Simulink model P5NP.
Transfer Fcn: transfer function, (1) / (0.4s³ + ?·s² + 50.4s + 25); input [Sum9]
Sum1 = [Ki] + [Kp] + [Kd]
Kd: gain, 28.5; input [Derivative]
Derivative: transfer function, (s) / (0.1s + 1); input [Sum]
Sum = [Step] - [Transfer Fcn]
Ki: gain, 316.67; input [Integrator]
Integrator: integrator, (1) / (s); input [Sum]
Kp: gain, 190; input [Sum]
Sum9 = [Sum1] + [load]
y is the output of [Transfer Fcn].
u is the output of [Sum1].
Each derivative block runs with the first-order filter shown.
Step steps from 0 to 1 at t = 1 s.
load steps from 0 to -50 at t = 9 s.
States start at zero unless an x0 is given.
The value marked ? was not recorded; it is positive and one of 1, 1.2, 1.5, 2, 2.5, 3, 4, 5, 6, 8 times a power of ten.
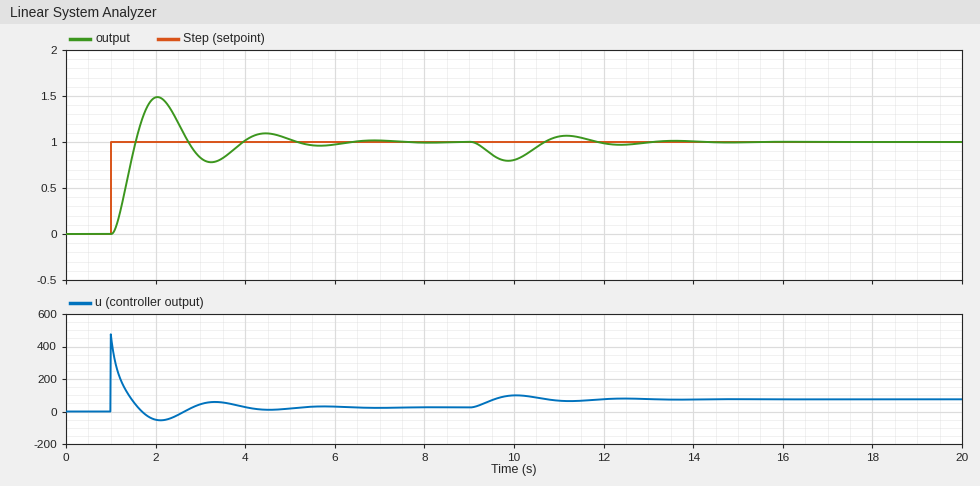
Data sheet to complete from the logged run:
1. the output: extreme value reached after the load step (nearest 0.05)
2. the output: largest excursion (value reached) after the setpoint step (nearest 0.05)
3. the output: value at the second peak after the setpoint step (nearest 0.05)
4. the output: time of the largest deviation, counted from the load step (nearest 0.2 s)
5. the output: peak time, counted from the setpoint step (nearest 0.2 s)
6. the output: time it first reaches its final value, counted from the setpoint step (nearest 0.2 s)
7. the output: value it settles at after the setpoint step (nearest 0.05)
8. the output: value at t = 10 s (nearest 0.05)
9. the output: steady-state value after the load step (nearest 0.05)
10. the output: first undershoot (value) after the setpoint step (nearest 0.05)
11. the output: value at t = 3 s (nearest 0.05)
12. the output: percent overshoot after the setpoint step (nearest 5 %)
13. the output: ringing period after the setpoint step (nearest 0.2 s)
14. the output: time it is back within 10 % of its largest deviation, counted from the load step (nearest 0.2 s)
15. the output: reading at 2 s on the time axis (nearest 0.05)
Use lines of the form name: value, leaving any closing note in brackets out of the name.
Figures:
the output: extreme value reached after the load step: 0.80
the output: largest excursion (value reached) after the setpoint step: 1.50
the output: value at the second peak after the setpoint step: 1.10
the output: time of the largest deviation, counted from the load step: 0.8 s
the output: peak time, counted from the setpoint step: 1.0 s
the output: time it first reaches its final value, counted from the setpoint step: 0.6 s
the output: value it settles at after the setpoint step: 1.00
the output: value at t = 10 s: 0.80
the output: steady-state value after the load step: 1.00
the output: first undershoot (value) after the setpoint step: 0.80
the output: value at t = 3 s: 0.85
the output: percent overshoot after the setpoint step: 50 %
the output: ringing period after the setpoint step: 2.4 s
the output: time it is back within 10 % of its largest deviation, counted from the load step: 3.8 s
the output: reading at 2 s on the time axis: 1.50
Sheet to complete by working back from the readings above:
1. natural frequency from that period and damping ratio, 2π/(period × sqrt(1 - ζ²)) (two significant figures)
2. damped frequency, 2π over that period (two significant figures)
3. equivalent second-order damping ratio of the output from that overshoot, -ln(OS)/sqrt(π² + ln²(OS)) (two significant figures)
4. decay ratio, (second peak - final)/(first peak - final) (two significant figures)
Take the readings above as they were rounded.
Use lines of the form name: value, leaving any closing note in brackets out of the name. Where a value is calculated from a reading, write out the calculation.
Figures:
natural frequency from that period and damping ratio, 2π/(period × sqrt(1 - ζ²)): 2π / (2.4 × sqrt(1 - 0.22²)) = 2.7 rad/s
damped frequency, 2π over that period: 2π / 2.4 = 2.6 rad/s
equivalent second-order damping ratio of the output from that overshoot, -ln(OS)/sqrt(π² + ln²(OS)): ln(0.5) = -0.693; 0.693 / sqrt(9.870 + 0.480) = 0.22
decay ratio, (second peak - final)/(first peak - final): (1.1 - 1) / (1.5 - 1) = 0.20
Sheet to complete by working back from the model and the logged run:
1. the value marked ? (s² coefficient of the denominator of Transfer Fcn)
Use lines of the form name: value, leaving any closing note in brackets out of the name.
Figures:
the value marked ?: 25
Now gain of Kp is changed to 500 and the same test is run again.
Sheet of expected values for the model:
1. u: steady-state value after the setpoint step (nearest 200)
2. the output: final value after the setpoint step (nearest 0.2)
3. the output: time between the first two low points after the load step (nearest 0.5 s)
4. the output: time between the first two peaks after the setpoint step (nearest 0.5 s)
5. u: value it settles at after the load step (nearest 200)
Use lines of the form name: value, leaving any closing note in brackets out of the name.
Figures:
u: steady-state value after the setpoint step: 0
the output: final value after the setpoint step: 1.0
the output: time between the first two low points after the load step: 1.5 s
the output: time between the first two peaks after the setpoint step: 1.5 s
u: value it settles at after the load step: 0
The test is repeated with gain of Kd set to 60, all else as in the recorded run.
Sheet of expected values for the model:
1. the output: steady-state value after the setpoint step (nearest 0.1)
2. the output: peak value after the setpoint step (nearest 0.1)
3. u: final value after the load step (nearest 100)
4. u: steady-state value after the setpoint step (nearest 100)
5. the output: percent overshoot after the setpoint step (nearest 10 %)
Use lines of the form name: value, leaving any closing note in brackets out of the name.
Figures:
the output: steady-state value after the setpoint step: 1.0
the output: peak value after the setpoint step: 1.3
u: final value after the load step: 100
u: steady-state value after the setpoint step: 0
the output: percent overshoot after the setpoint step: 30 %
